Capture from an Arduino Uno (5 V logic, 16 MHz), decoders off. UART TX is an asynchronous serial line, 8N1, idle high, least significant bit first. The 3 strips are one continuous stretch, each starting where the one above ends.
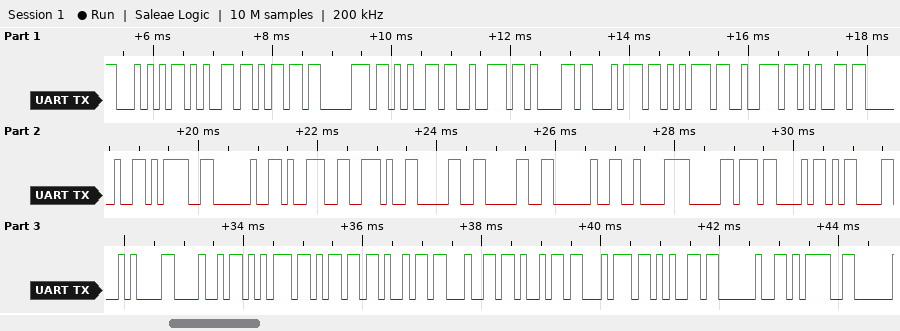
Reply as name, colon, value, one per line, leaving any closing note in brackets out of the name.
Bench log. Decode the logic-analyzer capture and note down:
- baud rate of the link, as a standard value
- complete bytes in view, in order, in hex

baud rate of the link, as a standard value: 9600 baud
complete bytes in view, in order, in hex: 0x54 0x65 0x6D 0x70 0x65 0x72 0x61 0x74 0x75 0x72 0x65 0x20 0x3D 0x20 0x39 0x2E 0x30 0x30 0x20 0xC2 0xB0 0x43 0x0D 0x0A 0x48 0x75 0x6D 0x69 0x64 0x69 0x74 0x65 0x20 0x3D
